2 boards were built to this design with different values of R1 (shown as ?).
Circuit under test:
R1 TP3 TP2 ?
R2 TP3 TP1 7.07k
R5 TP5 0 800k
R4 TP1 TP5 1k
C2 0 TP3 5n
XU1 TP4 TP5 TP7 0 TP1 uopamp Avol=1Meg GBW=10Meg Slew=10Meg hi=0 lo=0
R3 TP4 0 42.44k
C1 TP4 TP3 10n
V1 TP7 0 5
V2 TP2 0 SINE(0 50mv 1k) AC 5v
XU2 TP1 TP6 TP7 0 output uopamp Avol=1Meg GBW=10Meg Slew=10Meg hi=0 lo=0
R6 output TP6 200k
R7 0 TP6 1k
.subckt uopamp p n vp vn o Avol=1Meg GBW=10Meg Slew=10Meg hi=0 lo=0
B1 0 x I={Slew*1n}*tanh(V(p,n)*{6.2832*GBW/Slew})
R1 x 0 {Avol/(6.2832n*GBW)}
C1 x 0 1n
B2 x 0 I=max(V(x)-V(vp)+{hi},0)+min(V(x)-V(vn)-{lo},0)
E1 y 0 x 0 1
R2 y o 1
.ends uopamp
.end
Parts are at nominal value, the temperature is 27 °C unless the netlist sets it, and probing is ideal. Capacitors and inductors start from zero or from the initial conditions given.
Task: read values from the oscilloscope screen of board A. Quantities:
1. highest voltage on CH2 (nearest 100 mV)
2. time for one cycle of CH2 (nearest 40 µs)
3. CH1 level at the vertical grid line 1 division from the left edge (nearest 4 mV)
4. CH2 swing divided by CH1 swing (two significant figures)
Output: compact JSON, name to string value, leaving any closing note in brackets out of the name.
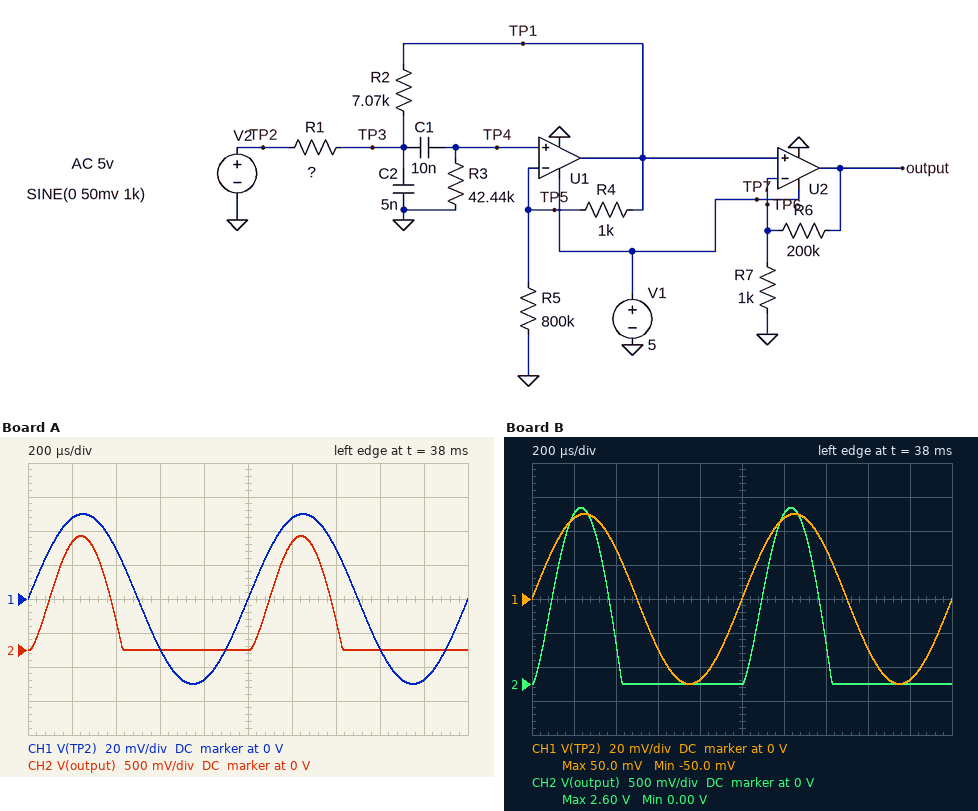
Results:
{"highest voltage on CH2": "1.7 V", "time for one cycle of CH2": "1.00 ms", "CH1 level at the vertical grid line 1 division from the left edge": "48 mV", "CH2 swing divided by CH1 swing": "17"}
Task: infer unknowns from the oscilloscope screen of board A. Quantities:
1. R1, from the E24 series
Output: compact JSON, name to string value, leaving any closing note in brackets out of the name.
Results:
{"R1, from the E24 series": "68 kΩ"}
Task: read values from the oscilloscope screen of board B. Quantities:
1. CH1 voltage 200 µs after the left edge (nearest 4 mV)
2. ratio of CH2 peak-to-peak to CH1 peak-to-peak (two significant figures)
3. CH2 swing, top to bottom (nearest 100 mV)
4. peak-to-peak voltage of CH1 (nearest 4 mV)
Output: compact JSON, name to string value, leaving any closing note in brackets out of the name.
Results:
{"CH1 voltage 200 µs after the left edge": "48 mV", "ratio of CH2 peak-to-peak to CH1 peak-to-peak": "26", "CH2 swing, top to bottom": "2.6 V", "peak-to-peak voltage of CH1": "100 mV"}
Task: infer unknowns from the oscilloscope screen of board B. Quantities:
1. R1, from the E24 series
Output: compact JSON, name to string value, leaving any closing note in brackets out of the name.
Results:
{"R1, from the E24 series": "39 kΩ"}
